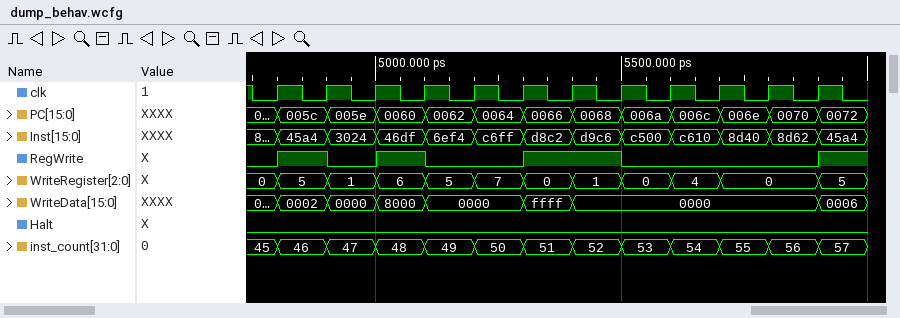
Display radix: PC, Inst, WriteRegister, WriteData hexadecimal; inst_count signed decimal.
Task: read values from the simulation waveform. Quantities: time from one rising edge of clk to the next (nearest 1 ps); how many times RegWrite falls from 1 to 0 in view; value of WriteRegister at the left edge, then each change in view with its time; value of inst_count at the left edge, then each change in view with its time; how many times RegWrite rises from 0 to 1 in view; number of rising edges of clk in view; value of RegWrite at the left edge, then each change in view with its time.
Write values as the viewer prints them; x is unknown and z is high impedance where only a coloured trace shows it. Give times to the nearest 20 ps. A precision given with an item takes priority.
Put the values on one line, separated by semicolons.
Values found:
100 ps; 3; 0, 5 at 4800 ps, 1 at 4900 ps, 6 at 5000 ps, 5 at 5100 ps, 7 at 5200 ps, 0 at 5300 ps, 1 at 5400 ps, 0 at 5500 ps, 4 at 5600 ps, 0 at 5700 ps, 5 at 5900 ps; 45, 46 at 4800 ps, 47 at 4900 ps, 48 at 5000 ps, 49 at 5100 ps, 50 at 5200 ps, 51 at 5300 ps, 52 at 5400 ps, 53 at 5500 ps, 54 at 5600 ps, 55 at 5700 ps, 56 at 5800 ps, 57 at 5900 ps; 4; 12; 0, 1 at 4800 ps, 0 at 4900 ps, 1 at 5000 ps, 0 at 5100 ps, 1 at 5300 ps, 0 at 5500 ps, 1 at 5900 ps
